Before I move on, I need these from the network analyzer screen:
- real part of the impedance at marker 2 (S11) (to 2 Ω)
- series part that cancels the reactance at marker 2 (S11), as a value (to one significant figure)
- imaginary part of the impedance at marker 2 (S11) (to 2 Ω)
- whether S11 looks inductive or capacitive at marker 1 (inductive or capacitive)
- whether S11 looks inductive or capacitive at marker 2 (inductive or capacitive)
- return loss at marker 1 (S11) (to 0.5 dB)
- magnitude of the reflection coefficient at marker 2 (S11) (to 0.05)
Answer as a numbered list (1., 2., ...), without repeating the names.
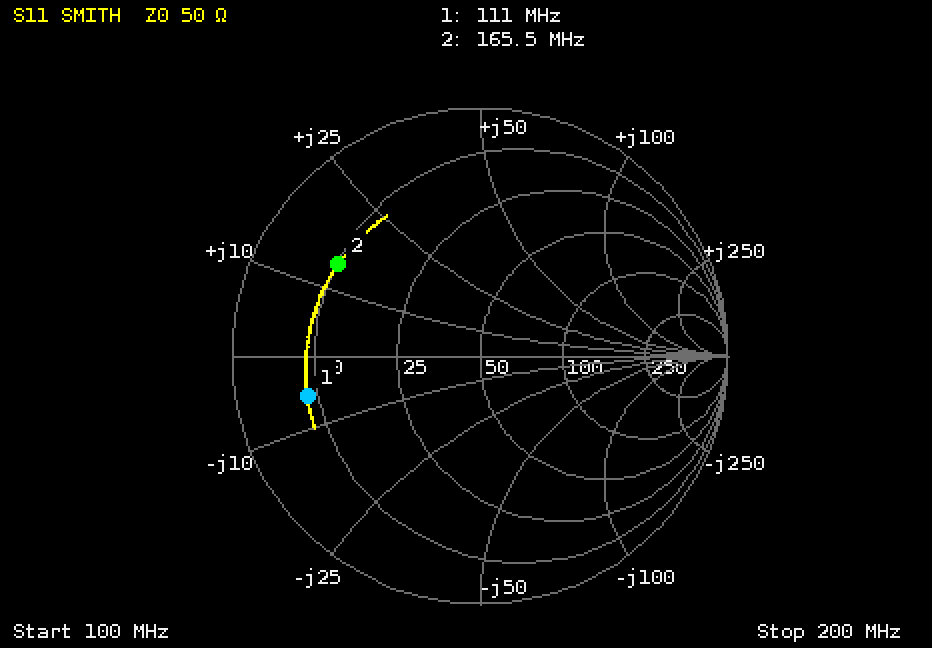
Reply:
1. 10 Ω
2. 70 pF
3. +14 Ω
4. capacitive
5. inductive
6. 3.0 dB
7. 0.70
